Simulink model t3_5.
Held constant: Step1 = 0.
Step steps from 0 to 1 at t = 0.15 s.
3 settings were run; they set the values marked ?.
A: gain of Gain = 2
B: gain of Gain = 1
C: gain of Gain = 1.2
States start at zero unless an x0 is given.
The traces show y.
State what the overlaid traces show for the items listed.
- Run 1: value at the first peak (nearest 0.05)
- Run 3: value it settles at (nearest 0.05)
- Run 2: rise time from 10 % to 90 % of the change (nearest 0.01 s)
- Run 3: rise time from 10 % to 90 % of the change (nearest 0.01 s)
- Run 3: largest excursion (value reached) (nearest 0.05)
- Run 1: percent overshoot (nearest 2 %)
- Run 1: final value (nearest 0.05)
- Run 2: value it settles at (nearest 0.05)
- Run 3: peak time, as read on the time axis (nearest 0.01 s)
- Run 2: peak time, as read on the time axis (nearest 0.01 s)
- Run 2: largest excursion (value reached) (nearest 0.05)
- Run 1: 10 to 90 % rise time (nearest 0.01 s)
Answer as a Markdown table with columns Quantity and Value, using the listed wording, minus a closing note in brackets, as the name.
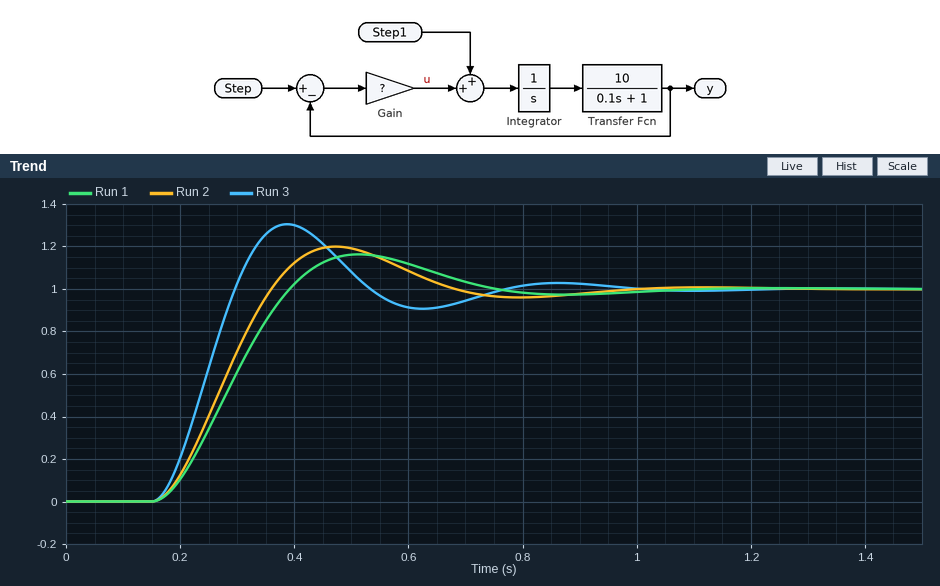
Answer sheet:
| Quantity | Value |
|---|---|
| Run 1: value at the first peak | 1.15 |
| Run 3: value it settles at | 1.00 |
| Run 2: rise time from 10 % to 90 % of the change | 0.14 s |
| Run 3: rise time from 10 % to 90 % of the change | 0.10 s |
| Run 3: largest excursion (value reached) | 1.30 |
| Run 1: percent overshoot | 16 % |
| Run 1: final value | 1.00 |
| Run 2: value it settles at | 1.00 |
| Run 3: peak time, as read on the time axis | 0.39 s |
| Run 2: peak time, as read on the time axis | 0.47 s |
| Run 2: largest excursion (value reached) | 1.20 |
| Run 1: 10 to 90 % rise time | 0.16 s |
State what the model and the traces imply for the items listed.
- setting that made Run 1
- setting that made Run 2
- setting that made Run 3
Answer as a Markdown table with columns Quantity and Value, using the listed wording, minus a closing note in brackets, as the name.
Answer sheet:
| Quantity | Value |
|---|---|
| setting that made Run 1 | B |
| setting that made Run 2 | C |
| setting that made Run 3 | A |
